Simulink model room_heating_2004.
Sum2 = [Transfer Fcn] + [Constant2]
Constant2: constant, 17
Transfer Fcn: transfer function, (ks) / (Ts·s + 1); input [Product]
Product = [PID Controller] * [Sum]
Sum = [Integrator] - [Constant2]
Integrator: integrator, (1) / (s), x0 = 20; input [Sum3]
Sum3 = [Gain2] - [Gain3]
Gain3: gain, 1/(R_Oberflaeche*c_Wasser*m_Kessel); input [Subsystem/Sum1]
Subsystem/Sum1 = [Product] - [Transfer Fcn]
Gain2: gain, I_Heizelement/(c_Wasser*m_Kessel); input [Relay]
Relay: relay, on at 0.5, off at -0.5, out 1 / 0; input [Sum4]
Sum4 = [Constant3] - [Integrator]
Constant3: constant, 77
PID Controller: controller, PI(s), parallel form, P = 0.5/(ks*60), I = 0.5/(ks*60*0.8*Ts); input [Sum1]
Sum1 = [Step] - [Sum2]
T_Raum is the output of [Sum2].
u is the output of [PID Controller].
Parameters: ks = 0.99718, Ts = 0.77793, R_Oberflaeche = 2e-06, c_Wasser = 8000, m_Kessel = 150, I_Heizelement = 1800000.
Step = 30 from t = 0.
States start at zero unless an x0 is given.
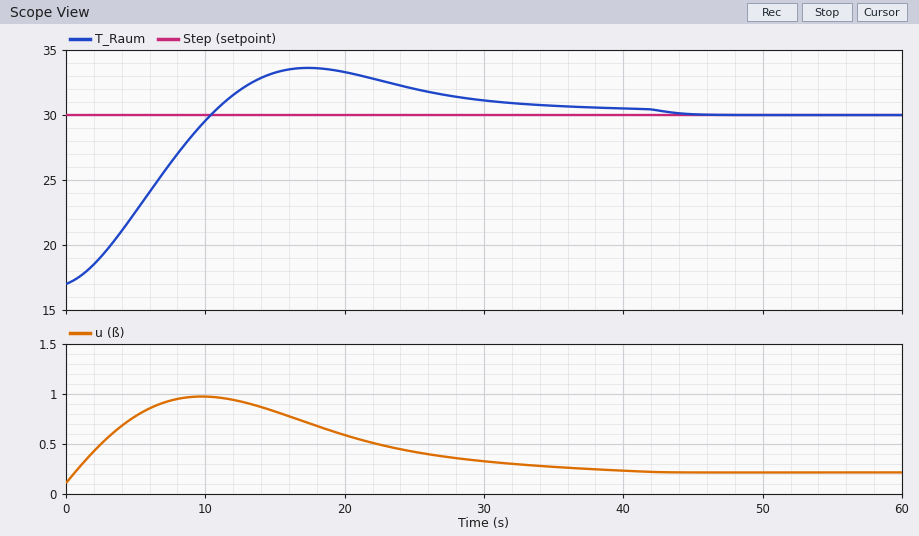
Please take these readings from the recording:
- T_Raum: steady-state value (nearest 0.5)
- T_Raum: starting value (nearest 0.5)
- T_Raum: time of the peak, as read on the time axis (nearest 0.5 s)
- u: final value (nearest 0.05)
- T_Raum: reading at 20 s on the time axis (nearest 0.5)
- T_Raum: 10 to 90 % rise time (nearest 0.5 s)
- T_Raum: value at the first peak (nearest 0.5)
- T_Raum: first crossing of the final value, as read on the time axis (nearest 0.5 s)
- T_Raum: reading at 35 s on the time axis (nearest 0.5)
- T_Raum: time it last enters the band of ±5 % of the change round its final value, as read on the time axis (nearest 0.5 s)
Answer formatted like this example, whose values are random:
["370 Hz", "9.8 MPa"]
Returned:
["30.0", "17.0", "17.5 s", "0.20", "33.5", "7.5 s", "33.5", "10.5 s", "30.5", "36.0 s"]
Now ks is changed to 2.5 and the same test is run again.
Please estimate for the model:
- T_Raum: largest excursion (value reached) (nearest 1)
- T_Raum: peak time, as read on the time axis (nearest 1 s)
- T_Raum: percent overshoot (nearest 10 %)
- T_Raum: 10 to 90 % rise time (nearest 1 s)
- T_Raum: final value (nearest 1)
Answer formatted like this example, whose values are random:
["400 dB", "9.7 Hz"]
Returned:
["37", "11 s", "50 %", "5 s", "30"]
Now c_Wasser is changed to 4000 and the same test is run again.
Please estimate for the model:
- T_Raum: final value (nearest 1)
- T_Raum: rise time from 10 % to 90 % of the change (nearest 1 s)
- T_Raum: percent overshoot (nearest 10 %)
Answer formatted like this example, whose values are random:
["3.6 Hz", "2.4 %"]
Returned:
["30", "6 s", "30 %"]
